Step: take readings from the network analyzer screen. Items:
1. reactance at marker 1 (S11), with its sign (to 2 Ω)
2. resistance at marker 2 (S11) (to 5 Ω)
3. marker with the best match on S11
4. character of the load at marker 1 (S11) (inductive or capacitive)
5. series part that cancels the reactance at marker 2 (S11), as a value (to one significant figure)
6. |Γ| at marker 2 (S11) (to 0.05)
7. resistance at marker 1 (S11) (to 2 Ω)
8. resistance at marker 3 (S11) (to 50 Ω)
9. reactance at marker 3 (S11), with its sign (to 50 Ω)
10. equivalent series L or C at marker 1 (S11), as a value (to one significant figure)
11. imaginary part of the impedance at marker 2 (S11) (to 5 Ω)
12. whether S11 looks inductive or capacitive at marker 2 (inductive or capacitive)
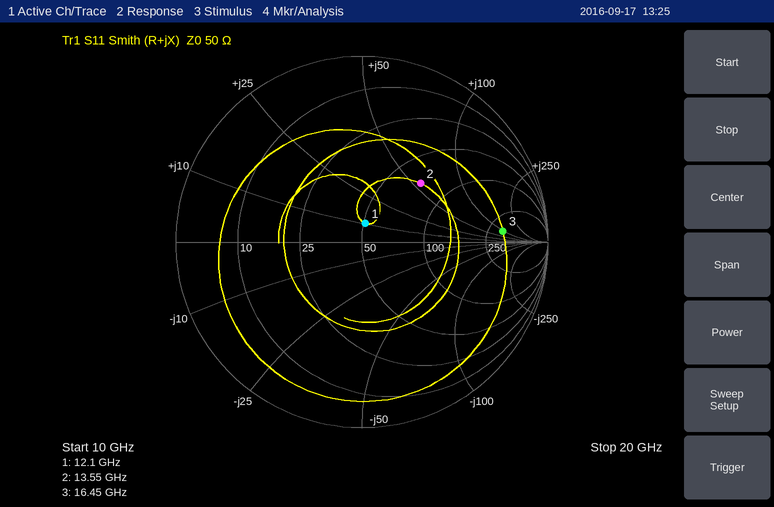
+10 Ω
70 Ω
marker 1
inductive
200 fF
0.45
50 Ω
350 Ω
+100 Ω
100 pH
+55 Ω
inductive
